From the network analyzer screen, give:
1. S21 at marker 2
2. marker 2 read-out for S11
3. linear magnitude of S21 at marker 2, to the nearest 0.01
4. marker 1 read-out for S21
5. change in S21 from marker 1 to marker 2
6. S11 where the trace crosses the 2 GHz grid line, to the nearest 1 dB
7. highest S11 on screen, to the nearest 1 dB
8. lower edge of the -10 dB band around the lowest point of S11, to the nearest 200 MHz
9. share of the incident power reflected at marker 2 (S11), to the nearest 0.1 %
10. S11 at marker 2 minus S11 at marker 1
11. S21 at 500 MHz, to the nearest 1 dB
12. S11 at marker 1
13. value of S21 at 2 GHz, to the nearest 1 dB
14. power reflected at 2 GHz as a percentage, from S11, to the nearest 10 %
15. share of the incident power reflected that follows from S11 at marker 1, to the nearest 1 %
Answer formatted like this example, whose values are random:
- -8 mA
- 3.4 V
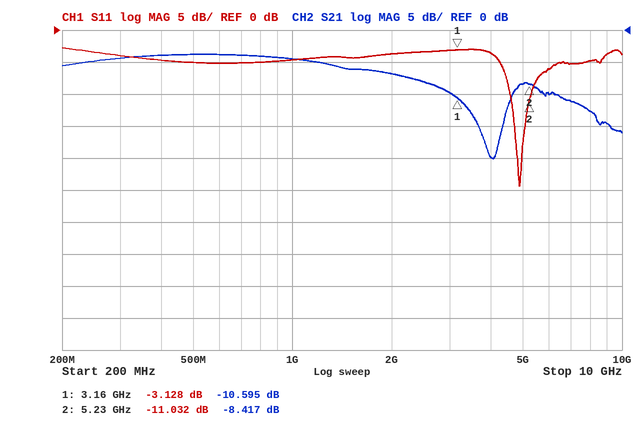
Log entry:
- -8.417 dB
- -11.032 dB
- 0.38
- -10.595 dB
- 2.178 dB
- -4 dB
- -3 dB
- 4.6 GHz
- 7.9 %
- -7.904 dB
- -4 dB
- -3.128 dB
- -7 dB
- 40 %
- 49 %
